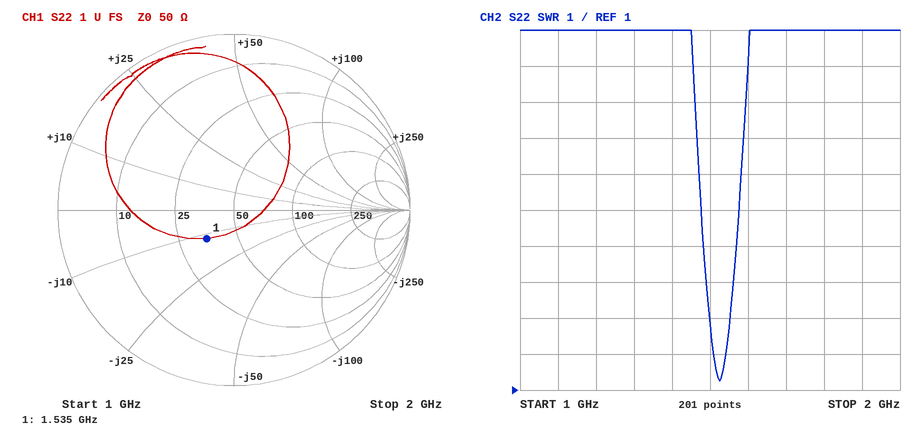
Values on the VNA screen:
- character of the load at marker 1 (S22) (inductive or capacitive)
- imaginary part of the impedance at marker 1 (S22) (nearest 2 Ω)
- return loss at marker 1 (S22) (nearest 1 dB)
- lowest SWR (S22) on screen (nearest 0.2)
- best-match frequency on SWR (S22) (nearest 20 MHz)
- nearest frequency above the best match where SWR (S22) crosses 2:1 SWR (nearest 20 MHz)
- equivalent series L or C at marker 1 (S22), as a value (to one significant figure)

capacitive
-12 Ω
13 dB
1.2
1.52 GHz
1.54 GHz
9 pF
